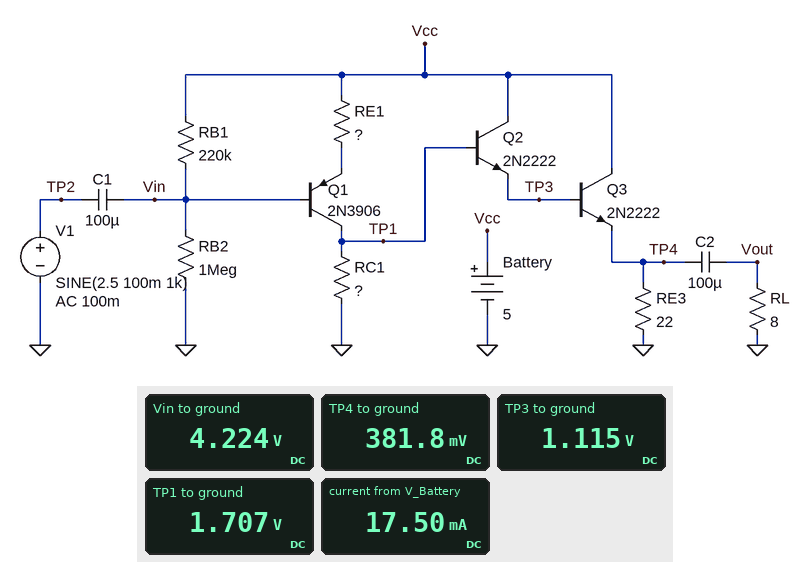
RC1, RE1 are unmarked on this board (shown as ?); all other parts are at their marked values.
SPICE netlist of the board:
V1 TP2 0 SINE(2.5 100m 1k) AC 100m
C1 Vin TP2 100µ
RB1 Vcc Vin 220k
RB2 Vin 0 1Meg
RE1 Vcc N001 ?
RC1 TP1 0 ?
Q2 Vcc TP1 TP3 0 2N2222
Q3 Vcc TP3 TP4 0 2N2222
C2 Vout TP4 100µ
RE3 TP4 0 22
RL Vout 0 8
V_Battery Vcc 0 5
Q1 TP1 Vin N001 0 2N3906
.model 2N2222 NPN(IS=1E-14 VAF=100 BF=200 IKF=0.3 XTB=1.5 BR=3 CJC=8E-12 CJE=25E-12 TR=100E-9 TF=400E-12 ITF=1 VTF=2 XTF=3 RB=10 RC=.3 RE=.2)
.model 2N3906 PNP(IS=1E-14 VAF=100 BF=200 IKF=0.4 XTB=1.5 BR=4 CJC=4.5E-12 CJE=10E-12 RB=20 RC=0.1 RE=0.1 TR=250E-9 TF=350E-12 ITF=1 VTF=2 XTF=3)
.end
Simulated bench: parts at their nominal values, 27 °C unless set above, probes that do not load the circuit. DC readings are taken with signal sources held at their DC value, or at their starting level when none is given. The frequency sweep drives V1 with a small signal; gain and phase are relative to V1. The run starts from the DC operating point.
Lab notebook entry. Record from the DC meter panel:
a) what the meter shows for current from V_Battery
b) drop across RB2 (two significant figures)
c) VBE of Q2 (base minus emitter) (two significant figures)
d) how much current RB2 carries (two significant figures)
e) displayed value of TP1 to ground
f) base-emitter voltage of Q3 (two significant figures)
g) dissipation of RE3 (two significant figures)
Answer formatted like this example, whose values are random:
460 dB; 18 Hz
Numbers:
17.50 mA; 4.2 V; 590 mV; 4.2 µA; 1.707 V; 730 mV; 6.6 mW
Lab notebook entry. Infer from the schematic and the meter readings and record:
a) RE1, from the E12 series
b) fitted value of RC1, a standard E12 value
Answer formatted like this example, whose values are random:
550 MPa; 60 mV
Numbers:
1.2 kΩ; 12 kΩ
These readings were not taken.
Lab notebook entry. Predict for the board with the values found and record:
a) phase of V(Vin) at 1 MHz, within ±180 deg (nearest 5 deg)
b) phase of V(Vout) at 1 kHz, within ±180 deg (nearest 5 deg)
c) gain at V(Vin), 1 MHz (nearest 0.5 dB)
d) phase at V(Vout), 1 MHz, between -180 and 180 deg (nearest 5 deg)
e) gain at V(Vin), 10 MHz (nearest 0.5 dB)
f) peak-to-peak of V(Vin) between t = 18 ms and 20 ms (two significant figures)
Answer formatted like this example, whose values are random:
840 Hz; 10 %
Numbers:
0 deg; -170 deg; 0 dB; 120 deg; 0 dB; 200 mV
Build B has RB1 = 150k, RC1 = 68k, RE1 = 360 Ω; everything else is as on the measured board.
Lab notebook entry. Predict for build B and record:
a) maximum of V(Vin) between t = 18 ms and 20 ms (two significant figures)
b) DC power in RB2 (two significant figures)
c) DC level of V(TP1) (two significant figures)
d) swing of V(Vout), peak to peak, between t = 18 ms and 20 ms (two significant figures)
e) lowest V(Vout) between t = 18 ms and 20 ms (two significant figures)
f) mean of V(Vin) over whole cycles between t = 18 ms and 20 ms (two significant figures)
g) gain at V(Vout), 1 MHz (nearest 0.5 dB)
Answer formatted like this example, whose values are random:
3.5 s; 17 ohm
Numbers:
4.5 V; 19 µW; 4.2 V; 1.7 V; -750 mV; 4.4 V; 23.0 dB
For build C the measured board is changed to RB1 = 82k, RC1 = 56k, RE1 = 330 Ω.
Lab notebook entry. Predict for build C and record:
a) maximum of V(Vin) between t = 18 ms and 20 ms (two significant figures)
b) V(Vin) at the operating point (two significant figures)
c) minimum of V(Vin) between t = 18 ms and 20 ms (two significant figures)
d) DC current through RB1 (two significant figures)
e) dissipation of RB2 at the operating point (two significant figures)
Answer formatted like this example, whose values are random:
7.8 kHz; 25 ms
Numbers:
4.7 V; 4.6 V; 4.5 V; 4.6 µA; 21 µW
